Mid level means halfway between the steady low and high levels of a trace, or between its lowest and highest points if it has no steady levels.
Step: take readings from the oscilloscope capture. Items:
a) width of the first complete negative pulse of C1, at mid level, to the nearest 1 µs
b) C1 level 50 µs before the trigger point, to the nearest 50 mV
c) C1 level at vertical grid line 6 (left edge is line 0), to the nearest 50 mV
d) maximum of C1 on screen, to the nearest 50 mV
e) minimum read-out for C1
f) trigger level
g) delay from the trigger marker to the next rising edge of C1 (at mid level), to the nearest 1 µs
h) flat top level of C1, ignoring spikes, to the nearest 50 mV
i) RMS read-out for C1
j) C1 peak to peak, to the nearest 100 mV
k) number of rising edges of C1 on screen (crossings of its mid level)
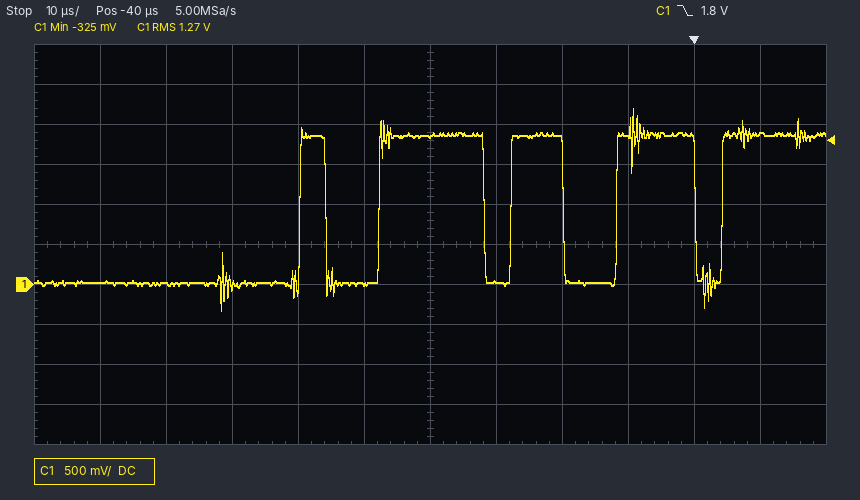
8 µs
0 mV
1.85 V
2.20 V
-325 mV
1.8 V
4 µs
1.85 V
1.27 V
2.50 V
5
